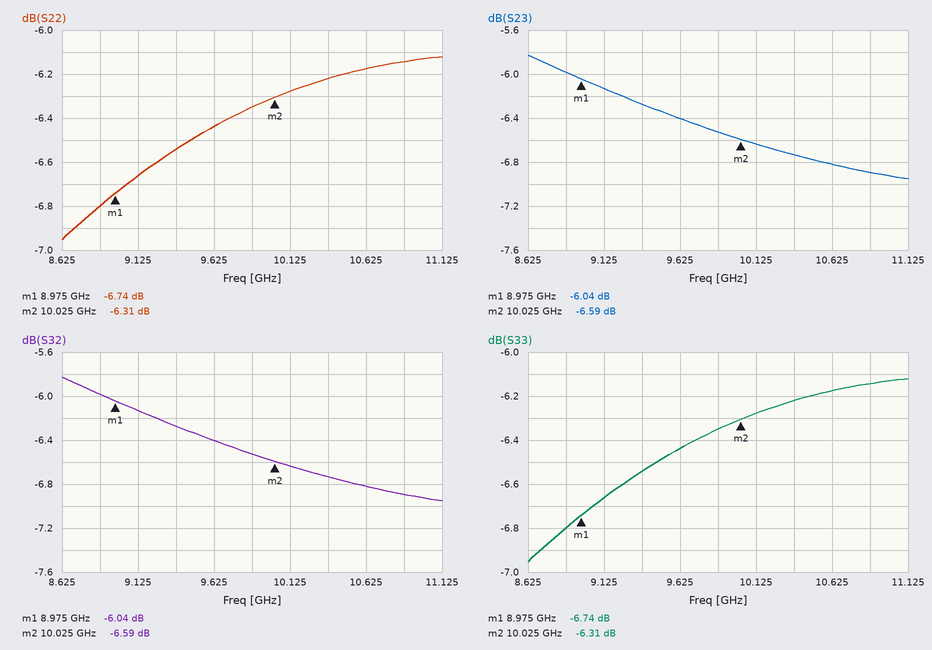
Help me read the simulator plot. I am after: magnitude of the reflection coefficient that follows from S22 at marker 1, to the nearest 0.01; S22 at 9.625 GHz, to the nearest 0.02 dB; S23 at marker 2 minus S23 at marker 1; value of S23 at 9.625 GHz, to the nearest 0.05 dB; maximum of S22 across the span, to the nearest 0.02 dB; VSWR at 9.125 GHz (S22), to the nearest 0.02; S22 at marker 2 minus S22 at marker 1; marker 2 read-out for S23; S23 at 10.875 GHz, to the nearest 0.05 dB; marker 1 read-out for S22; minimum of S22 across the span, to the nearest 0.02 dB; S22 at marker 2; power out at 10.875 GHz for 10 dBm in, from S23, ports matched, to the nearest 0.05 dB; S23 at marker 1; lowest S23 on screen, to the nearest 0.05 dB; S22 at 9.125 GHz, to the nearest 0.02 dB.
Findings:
0.46
-6.44 dB
-0.55 dB
-6.40 dB
-6.12 dB
2.74
0.43 dB
-6.59 dB
-6.90 dB
-6.74 dB
-6.96 dB
-6.31 dB
3.10 dBm
-6.04 dB
-6.95 dB
-6.66 dB
